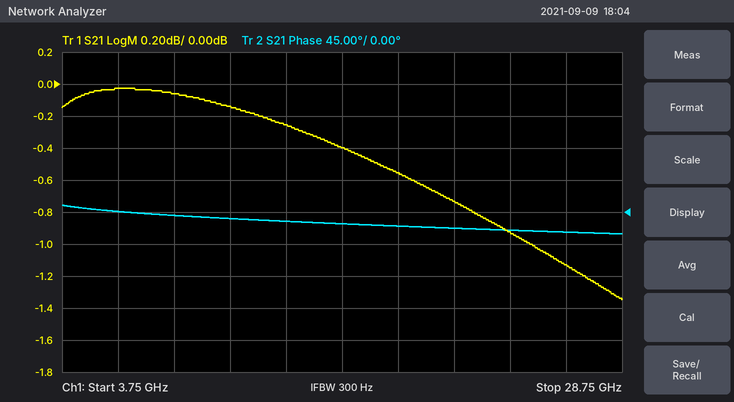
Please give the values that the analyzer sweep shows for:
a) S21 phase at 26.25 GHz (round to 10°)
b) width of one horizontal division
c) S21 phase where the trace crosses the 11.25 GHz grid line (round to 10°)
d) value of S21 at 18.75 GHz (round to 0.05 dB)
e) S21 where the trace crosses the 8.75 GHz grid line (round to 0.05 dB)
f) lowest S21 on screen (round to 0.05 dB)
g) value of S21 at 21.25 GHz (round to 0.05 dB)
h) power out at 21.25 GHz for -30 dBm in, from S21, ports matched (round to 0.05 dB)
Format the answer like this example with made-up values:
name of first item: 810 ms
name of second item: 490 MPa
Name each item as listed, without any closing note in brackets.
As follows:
S21 phase at 26.25 GHz: -30°
width of one horizontal division: 2.5 GHz
S21 phase where the trace crosses the 11.25 GHz grid line: -10°
value of S21 at 18.75 GHz: -0.55 dB
S21 where the trace crosses the 8.75 GHz grid line: -0.05 dB
lowest S21 on screen: -1.35 dB
value of S21 at 21.25 GHz: -0.75 dB
power out at 21.25 GHz for -30 dBm in, from S21, ports matched: -30.75 dBm
